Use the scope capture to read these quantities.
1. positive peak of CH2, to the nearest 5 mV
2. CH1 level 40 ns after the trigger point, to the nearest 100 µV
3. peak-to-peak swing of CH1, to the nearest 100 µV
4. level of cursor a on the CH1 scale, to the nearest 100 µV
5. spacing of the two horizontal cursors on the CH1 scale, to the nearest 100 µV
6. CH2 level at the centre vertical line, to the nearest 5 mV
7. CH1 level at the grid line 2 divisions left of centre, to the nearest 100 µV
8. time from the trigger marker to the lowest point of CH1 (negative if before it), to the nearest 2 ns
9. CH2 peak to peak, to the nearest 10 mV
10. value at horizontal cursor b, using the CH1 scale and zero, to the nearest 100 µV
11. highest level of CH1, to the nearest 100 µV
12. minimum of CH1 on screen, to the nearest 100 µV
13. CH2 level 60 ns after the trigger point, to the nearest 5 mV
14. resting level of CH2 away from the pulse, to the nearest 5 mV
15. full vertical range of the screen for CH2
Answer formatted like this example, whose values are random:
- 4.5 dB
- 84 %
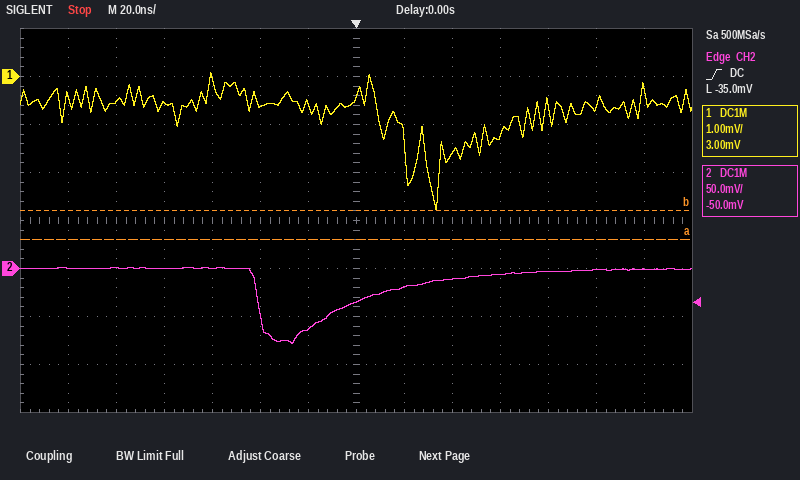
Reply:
- 0 mV
- -1.6 mV
- 2.9 mV
- -3.4 mV
- 600 µV
- -35 mV
- -600 µV
- +34 ns
- 80 mV
- -2.8 mV
- 100 µV
- -2.8 mV
- -5 mV
- 0 mV
- 400 mV
